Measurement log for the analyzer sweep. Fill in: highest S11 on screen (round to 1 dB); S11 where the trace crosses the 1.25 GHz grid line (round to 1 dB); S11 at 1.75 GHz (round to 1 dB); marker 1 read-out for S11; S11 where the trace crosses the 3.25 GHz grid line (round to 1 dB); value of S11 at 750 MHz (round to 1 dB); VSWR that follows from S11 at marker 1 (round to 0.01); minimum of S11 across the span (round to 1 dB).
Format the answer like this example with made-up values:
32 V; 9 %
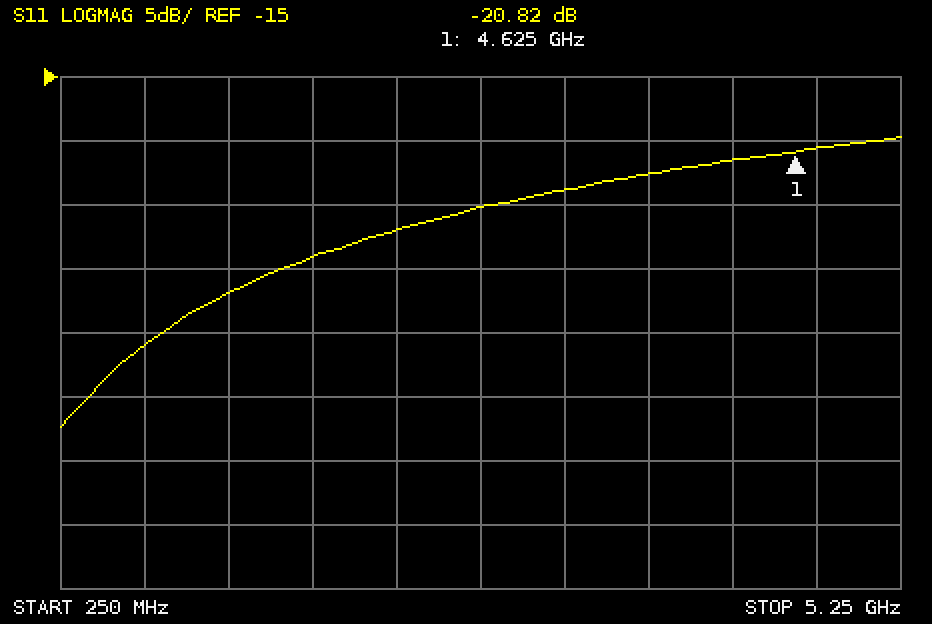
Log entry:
-20 dB; -32 dB; -29 dB; -20.82 dB; -24 dB; -36 dB; 1.20; -42 dB
